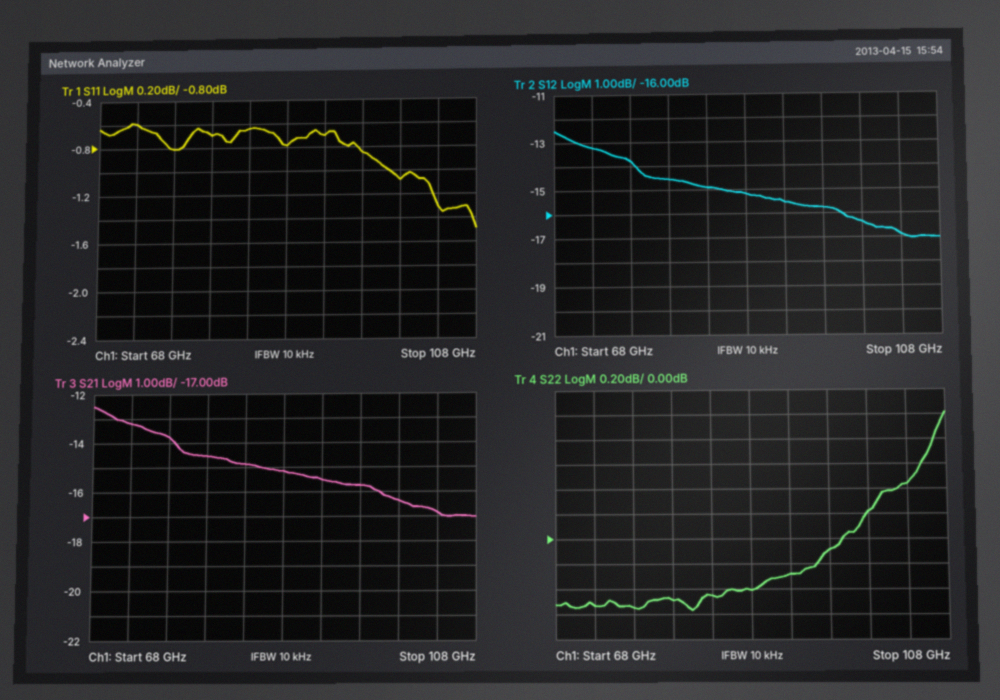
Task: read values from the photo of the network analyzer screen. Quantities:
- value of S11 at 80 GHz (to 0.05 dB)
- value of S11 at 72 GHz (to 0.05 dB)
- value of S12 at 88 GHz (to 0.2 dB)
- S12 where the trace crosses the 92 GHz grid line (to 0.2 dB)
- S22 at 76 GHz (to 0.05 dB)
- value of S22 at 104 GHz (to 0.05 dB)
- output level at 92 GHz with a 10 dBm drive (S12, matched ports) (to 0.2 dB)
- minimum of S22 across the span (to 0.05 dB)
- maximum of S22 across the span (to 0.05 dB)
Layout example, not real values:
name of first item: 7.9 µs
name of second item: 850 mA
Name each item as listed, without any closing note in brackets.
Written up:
value of S11 at 80 GHz: -0.70 dB
value of S11 at 72 GHz: -0.60 dB
value of S12 at 88 GHz: -15.2 dB
S12 where the trace crosses the 92 GHz grid line: -15.6 dB
S22 at 76 GHz: -0.55 dB
value of S22 at 104 GHz: 0.45 dB
output level at 92 GHz with a 10 dBm drive (S12, matched ports): -5.6 dBm
minimum of S22 across the span: -0.55 dB
maximum of S22 across the span: 1.00 dB
